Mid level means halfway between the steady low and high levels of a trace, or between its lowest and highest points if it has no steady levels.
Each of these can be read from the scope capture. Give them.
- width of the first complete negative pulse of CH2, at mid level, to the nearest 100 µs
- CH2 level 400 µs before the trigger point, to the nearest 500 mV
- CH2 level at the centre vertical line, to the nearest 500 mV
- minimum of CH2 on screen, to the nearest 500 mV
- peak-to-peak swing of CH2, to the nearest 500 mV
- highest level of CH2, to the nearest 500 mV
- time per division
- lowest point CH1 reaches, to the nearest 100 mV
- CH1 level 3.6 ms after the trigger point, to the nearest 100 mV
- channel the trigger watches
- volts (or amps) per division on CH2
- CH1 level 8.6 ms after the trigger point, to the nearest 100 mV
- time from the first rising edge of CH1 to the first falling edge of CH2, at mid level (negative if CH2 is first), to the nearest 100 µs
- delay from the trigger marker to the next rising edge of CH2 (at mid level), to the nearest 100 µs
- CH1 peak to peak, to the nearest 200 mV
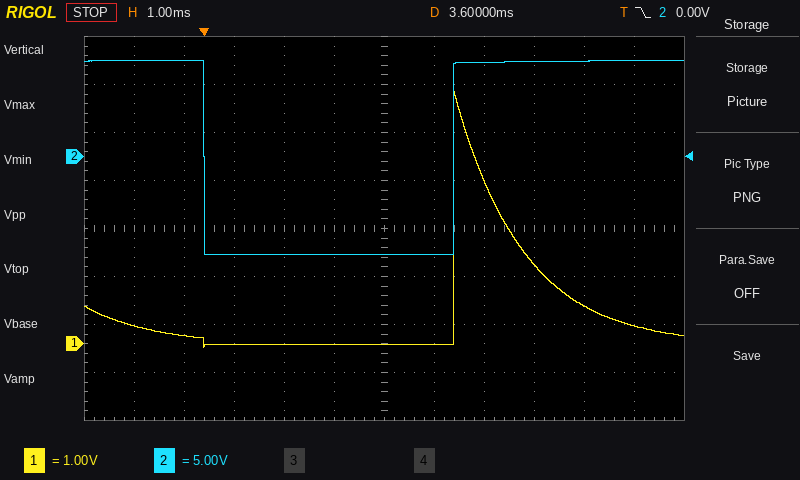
5.0 ms
10.0 V
-10.0 V
-10.0 V
20.0 V
10.0 V
1 ms
-100 mV
0.0 V
CH2
5 V
400 mV
-5.0 ms
5.0 ms
5.4 V
